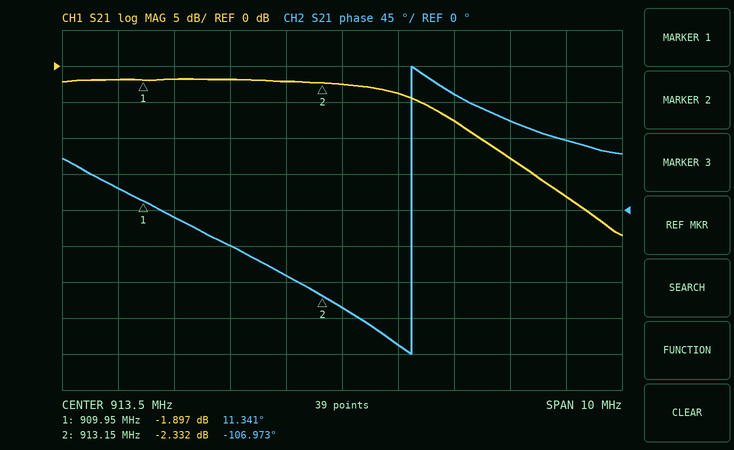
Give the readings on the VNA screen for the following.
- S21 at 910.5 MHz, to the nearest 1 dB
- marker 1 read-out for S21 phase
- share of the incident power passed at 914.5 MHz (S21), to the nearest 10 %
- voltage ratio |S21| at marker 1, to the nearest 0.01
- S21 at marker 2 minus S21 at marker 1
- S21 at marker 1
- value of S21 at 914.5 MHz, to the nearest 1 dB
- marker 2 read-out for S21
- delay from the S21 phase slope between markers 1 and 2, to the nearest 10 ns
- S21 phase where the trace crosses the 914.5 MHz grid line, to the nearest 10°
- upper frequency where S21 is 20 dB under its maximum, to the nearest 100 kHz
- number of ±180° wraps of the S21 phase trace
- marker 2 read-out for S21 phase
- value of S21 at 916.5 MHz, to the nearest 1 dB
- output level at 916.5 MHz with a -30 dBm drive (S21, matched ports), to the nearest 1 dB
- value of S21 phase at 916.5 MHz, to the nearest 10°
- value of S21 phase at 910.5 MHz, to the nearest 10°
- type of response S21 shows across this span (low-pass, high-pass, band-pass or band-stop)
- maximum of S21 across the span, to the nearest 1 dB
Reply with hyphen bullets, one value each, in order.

- -2 dB
- 11.341°
- 40 %
- 0.80
- -0.435 dB
- -1.897 dB
- -4 dB
- -2.332 dB
- 100 ns
- -170°
- 918.2 MHz
- 1
- -106.973°
- -13 dB
- -43 dBm
- 110°
- -10°
- low-pass
- -2 dB
